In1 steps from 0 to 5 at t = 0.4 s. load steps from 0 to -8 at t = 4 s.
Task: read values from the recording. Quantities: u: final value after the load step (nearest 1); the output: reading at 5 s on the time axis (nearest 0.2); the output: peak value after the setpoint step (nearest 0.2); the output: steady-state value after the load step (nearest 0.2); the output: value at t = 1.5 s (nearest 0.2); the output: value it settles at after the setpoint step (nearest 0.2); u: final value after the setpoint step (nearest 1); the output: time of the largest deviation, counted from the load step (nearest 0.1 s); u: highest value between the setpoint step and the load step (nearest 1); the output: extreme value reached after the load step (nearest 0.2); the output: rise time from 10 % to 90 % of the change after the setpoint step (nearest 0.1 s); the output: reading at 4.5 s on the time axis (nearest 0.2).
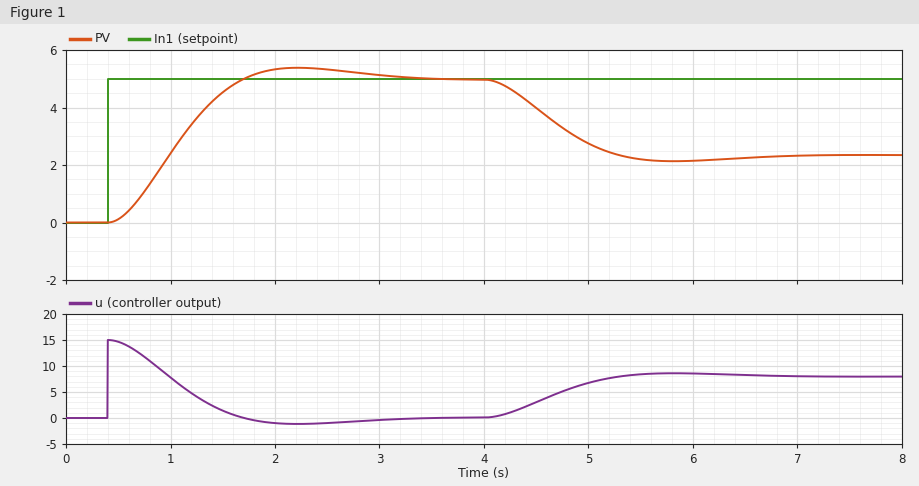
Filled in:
8
2.8
5.4
2.4
4.6
5.0
0
1.8 s
15
2.2
0.9 s
4.0
